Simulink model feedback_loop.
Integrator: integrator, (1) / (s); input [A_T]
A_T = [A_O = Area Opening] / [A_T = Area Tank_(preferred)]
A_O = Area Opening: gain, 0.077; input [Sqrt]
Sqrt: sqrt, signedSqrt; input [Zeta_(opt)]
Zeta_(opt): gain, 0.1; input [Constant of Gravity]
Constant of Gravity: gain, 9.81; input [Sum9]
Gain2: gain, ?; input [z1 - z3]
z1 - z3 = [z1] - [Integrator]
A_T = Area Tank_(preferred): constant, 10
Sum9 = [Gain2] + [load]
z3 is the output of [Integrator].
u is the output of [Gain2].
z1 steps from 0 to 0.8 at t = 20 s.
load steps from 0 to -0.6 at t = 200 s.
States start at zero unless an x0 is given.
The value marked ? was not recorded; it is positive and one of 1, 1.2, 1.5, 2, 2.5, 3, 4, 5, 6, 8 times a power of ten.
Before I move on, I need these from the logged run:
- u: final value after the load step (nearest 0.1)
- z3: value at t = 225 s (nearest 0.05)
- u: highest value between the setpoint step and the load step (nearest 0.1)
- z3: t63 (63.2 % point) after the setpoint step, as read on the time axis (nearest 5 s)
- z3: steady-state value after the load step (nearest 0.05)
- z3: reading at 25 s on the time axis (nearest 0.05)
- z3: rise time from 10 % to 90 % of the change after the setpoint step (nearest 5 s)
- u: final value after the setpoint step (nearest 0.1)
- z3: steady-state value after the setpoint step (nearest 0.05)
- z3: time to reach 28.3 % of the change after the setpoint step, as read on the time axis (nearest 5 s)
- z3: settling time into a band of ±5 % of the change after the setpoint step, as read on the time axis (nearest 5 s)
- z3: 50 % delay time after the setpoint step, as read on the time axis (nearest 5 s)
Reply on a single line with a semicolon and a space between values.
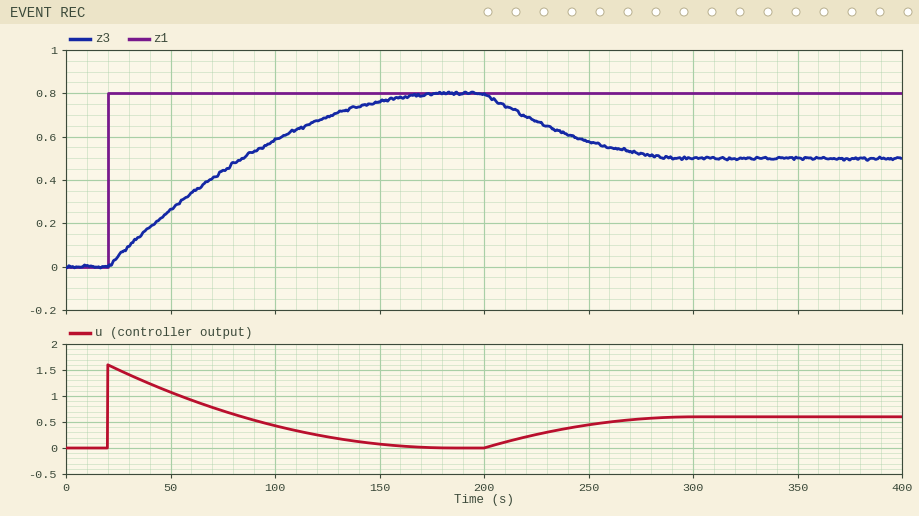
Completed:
0.6; 0.65; 1.6; 85 s; 0.50; 0.05; 105 s; 0.0; 0.80; 45 s; 150 s; 70 s
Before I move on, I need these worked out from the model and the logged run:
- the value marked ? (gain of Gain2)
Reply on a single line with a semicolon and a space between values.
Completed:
2
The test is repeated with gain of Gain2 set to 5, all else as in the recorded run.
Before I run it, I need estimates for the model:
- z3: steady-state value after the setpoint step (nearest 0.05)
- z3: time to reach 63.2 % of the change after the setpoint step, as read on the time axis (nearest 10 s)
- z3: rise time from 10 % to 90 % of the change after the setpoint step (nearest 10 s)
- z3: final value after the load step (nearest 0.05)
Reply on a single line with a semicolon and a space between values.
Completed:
0.80; 60 s; 70 s; 0.70
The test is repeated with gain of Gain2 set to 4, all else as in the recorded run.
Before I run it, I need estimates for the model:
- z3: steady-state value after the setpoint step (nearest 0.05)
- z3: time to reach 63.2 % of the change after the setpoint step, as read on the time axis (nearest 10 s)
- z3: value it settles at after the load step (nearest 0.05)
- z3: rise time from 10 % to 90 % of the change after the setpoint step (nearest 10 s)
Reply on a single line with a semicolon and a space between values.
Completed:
0.80; 70 s; 0.65; 70 s
